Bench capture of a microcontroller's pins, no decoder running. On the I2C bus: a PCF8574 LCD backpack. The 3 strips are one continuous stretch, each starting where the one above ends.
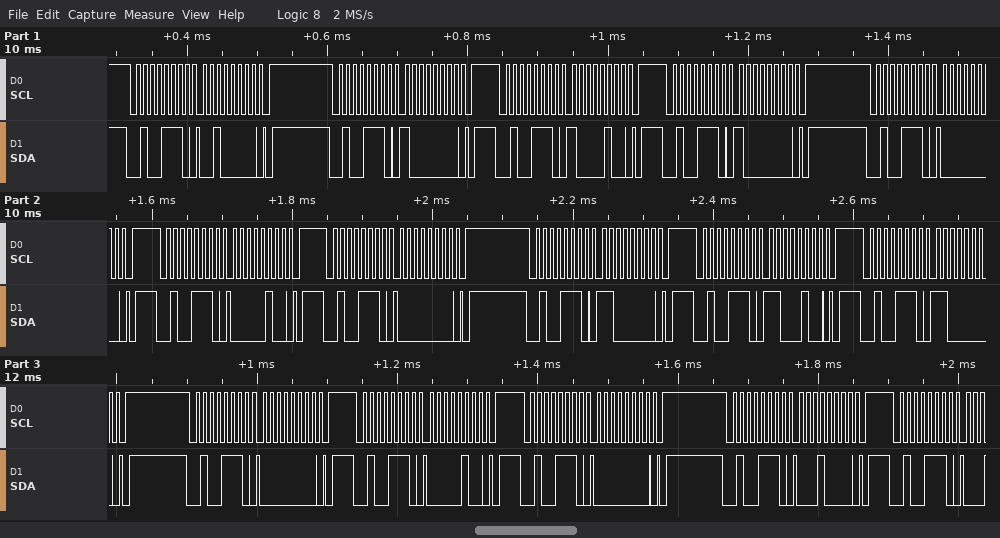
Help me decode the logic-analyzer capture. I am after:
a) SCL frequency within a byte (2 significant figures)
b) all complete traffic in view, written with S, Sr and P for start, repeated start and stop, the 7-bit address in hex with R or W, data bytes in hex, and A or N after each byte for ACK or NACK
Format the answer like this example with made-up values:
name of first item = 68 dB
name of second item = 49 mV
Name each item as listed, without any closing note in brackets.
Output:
SCL frequency within a byte = 100 kHz
all complete traffic in view, written with S, Sr and P for start, repeated start and stop, the 7-bit address in hex with R or W, data bytes in hex, and A or N after each byte for ACK or NACK = S 27W A 20 A P S 27W A 80 A P S 27W A 84 A P S 27W A 80 A P S 27W A 00 A P S 27W A 04 A P S 27W A 00 A P S 27W A C0 A P S 27W A C4 A P S 27W A C0 A P S 27W A 00 A P S 27W A 04 A P S 27W A 00 A P S 27W A 10 A P S 27W A
